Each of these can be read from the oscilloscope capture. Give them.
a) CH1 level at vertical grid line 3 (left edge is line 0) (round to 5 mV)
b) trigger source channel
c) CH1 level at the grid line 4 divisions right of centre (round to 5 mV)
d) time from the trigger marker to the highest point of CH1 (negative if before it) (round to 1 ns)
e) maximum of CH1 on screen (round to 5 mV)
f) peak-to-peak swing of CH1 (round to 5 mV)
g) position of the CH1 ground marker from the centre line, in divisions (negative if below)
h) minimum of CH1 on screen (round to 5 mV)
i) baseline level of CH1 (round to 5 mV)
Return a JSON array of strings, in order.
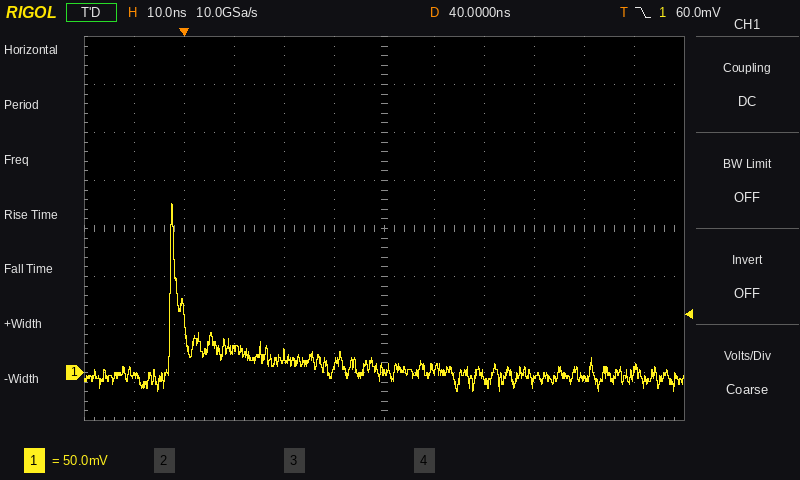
["25 mV", "CH1", "-5 mV", "-2 ns", "175 mV", "195 mV", "-3.0 div", "-20 mV", "0 mV"]
